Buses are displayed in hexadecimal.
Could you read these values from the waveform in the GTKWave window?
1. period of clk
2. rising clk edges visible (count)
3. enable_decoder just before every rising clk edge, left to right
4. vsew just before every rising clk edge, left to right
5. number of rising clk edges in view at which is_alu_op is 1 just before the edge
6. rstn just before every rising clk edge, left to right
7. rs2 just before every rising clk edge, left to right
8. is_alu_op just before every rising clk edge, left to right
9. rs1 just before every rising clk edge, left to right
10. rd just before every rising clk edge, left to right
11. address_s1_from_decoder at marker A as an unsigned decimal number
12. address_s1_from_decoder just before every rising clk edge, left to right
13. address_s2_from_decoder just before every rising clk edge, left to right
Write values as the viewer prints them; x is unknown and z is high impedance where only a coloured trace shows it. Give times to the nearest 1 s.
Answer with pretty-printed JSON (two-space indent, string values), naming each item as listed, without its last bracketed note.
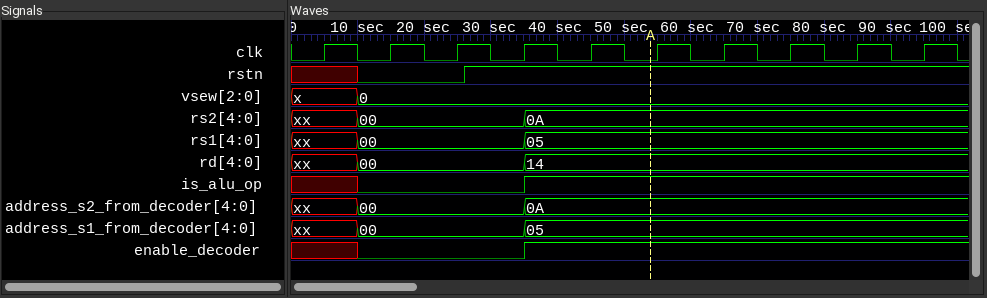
{
  "period of clk": "10 s",
  "rising clk edges visible": "10",
  "enable_decoder just before every rising clk edge, left to right": "x 0 0 0 1 1 1 1 1 1",
  "vsew just before every rising clk edge, left to right": "x, 0, 0, 0, 0, 0, 0, 0, 0, 0",
  "number of rising clk edges in view at which is_alu_op is 1 just before the edge": "6",
  "rstn just before every rising clk edge, left to right": "x 0 0 1 1 1 1 1 1 1",
  "rs2 just before every rising clk edge, left to right": "xx, 00, 00, 00, 0A, 0A, 0A, 0A, 0A, 0A",
  "is_alu_op just before every rising clk edge, left to right": "x 0 0 0 1 1 1 1 1 1",
  "rs1 just before every rising clk edge, left to right": "xx, 00, 00, 00, 05, 05, 05, 05, 05, 05",
  "rd just before every rising clk edge, left to right": "xx, 00, 00, 00, 14, 14, 14, 14, 14, 14",
  "address_s1_from_decoder at marker A as an unsigned decimal number": "5",
  "address_s1_from_decoder just before every rising clk edge, left to right": "xx, 00, 00, 00, 05, 05, 05, 05, 05, 05",
  "address_s2_from_decoder just before every rising clk edge, left to right": "xx, 00, 00, 00, 0A, 0A, 0A, 0A, 0A, 0A"
}
